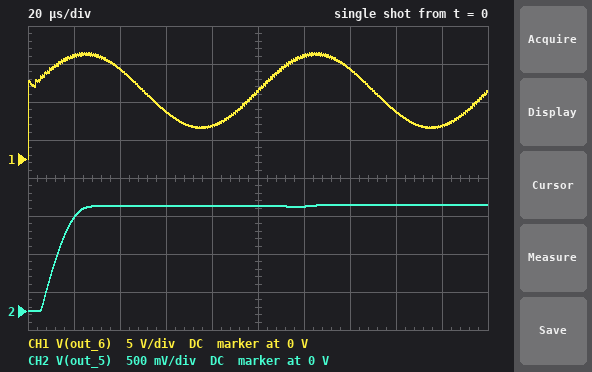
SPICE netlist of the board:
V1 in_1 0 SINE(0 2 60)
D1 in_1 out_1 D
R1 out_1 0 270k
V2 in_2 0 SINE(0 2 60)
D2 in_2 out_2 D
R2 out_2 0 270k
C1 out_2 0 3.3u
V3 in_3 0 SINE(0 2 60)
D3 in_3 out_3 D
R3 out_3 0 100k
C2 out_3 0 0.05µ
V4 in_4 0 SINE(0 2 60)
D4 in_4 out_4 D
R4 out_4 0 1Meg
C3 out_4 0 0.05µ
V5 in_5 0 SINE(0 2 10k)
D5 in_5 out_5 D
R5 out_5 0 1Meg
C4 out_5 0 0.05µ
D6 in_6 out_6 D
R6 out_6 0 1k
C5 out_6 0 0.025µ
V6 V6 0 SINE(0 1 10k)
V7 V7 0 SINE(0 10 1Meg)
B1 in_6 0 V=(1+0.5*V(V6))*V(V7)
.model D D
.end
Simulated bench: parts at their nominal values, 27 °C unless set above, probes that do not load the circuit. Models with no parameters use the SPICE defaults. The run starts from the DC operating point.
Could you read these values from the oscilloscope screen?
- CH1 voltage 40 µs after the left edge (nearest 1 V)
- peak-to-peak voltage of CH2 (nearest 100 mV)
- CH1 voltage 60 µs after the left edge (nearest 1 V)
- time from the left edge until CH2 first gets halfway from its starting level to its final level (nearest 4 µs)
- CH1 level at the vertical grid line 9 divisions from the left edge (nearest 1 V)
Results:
12 V
1.4 V
6 V
12 µs
4 V
